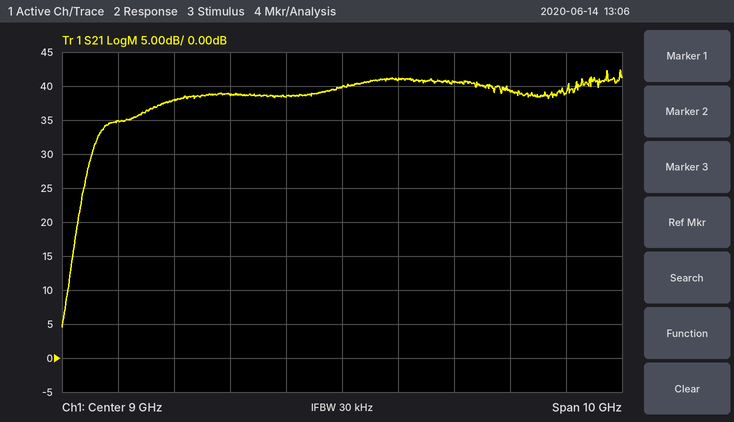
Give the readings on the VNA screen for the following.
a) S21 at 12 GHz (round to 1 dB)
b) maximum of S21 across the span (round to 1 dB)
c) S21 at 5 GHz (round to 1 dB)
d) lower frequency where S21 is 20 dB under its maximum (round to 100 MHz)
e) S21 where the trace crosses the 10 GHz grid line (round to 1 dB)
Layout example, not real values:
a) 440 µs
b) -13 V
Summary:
a) 39 dB
b) 42 dB
c) 35 dB
d) 4.3 GHz
e) 41 dB
